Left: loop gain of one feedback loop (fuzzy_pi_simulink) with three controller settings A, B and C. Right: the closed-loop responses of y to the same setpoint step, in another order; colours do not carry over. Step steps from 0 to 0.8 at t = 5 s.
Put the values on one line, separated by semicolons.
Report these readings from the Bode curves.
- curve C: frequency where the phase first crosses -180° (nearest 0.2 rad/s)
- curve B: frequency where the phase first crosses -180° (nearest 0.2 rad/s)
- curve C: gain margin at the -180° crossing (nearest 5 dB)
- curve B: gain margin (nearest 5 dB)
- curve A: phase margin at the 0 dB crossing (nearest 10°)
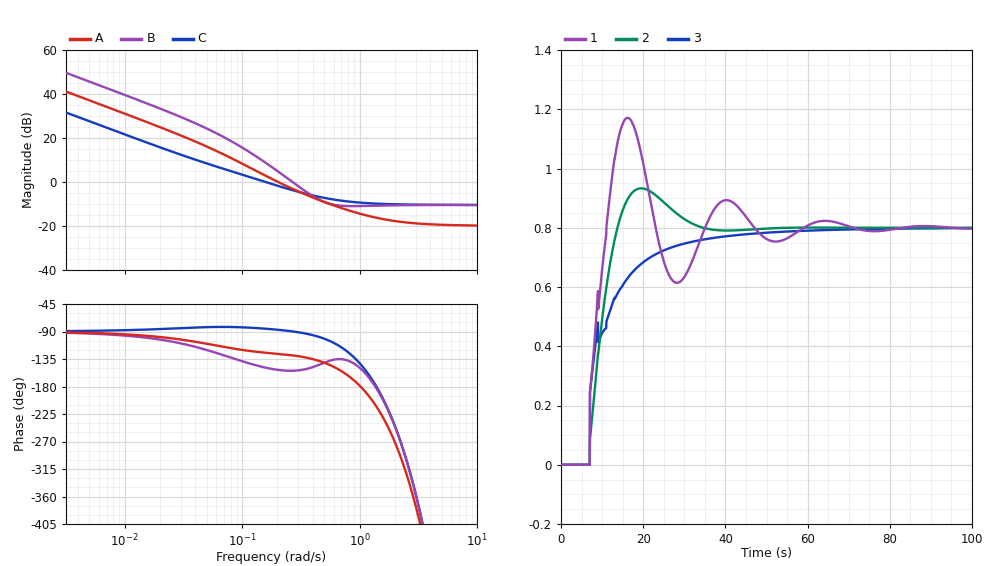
1.4 rad/s; 1.4 rad/s; 10 dB; 10 dB; 50°
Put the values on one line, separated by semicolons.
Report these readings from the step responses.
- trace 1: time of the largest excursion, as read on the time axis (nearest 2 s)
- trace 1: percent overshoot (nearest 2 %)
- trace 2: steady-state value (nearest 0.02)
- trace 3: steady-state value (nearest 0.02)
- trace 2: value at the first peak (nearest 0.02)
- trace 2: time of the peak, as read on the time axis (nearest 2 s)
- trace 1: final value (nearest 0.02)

16 s; 46 %; 0.80; 0.80; 0.94; 20 s; 0.80
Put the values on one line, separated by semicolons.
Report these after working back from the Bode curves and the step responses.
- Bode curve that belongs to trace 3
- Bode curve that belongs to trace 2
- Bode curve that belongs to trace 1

C; A; B
